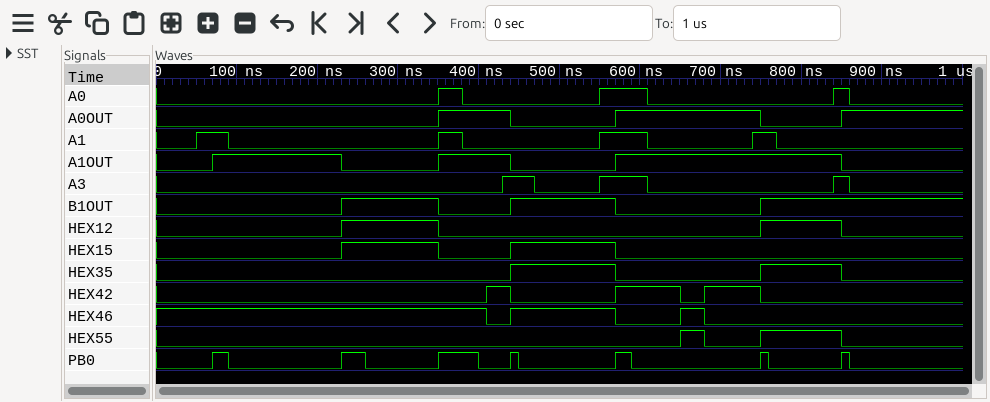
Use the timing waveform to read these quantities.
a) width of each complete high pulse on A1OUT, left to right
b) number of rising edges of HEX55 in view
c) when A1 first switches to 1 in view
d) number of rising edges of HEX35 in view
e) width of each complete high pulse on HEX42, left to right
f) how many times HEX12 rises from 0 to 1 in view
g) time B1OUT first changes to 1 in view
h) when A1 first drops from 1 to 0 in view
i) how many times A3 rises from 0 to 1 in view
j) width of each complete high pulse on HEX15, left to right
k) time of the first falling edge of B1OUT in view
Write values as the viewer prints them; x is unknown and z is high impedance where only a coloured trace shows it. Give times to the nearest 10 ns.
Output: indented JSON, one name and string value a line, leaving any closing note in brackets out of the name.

{
  "width of each complete high pulse on A1OUT, left to right": "160 ns, 90 ns, 280 ns",
  "number of rising edges of HEX55 in view": "2",
  "when A1 first switches to 1 in view": "50 ns",
  "number of rising edges of HEX35 in view": "2",
  "width of each complete high pulse on HEX42, left to right": "30 ns, 80 ns, 70 ns",
  "how many times HEX12 rises from 0 to 1 in view": "2",
  "time B1OUT first changes to 1 in view": "230 ns",
  "when A1 first drops from 1 to 0 in view": "90 ns",
  "how many times A3 rises from 0 to 1 in view": "3",
  "width of each complete high pulse on HEX15, left to right": "120 ns, 130 ns",
  "time of the first falling edge of B1OUT in view": "350 ns"
}
